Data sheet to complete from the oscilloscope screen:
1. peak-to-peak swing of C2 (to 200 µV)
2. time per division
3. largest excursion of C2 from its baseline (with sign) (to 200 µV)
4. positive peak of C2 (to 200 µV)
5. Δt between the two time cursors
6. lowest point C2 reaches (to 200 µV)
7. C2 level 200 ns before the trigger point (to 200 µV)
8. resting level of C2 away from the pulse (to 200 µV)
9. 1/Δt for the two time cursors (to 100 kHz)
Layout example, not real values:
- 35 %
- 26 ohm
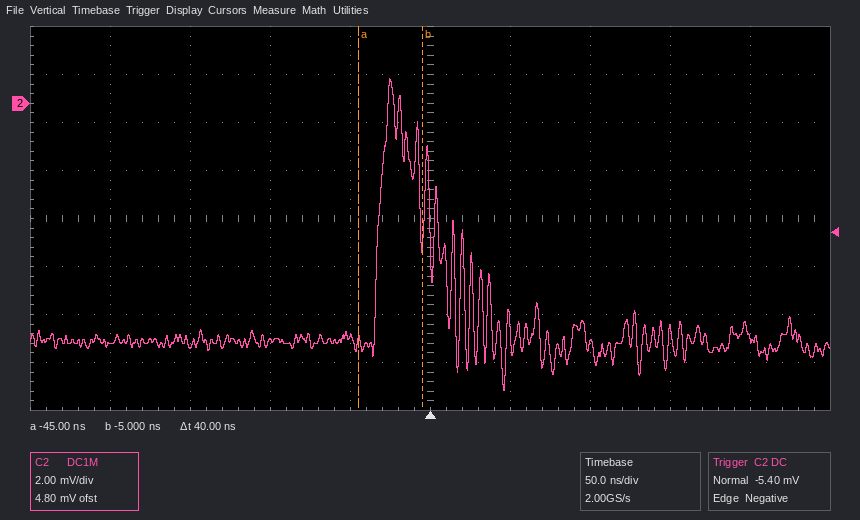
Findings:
- 13.0 mV
- 50 ns
- +11.0 mV
- 1.0 mV
- 40 ns
- -12.0 mV
- -10.0 mV
- -10.0 mV
- 25.0 MHz
